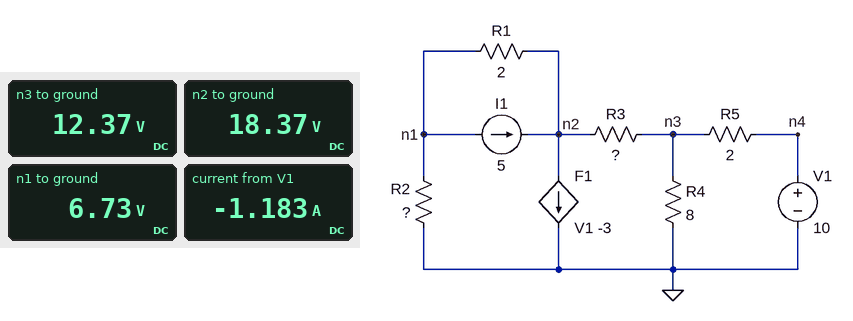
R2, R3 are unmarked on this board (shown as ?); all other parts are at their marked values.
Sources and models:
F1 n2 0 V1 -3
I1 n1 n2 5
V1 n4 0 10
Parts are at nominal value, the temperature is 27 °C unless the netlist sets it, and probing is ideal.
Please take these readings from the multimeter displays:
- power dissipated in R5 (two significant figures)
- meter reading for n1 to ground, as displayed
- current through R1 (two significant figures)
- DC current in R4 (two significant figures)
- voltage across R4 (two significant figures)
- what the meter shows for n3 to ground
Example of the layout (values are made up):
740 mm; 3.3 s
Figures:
2.8 W; 6.73 V; 5.8 A; 1.5 A; 12 V; 12.37 V
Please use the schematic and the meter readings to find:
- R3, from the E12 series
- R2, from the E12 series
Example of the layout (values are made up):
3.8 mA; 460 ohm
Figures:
2.2 Ω; 8.2 Ω
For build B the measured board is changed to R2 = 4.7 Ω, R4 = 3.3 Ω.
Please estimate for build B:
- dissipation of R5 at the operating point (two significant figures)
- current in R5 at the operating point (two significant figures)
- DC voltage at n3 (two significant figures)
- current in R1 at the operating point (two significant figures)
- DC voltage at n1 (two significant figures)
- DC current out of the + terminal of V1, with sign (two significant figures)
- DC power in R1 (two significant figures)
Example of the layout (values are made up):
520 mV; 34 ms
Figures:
100 W; 7.1 A; 24 V; 12 A; 32 V; -7.1 A; 280 W
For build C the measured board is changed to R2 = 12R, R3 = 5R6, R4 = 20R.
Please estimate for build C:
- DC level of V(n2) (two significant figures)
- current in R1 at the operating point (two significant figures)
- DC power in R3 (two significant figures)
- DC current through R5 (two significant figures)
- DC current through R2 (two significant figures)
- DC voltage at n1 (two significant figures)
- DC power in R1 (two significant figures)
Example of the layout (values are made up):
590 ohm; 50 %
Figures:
17 V; 5.5 A; 6.6 W; 530 mA; 510 mA; 6.1 V; 61 W
